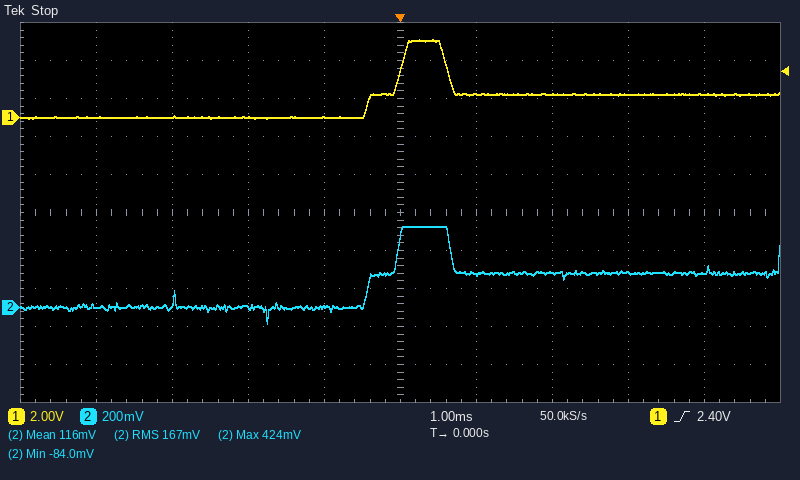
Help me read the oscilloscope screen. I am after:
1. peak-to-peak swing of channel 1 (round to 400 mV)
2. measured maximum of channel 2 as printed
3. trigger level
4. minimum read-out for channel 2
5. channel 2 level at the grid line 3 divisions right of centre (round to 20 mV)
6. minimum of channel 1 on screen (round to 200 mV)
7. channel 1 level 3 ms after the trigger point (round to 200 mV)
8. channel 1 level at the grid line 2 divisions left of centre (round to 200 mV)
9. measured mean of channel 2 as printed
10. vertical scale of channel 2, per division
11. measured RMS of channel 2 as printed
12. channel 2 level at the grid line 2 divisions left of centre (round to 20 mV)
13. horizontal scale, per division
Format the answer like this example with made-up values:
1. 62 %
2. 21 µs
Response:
1. 4.0 V
2. 424 mV
3. 2.40 V
4. -84.0 mV
5. 180 mV
6. 0.0 V
7. 1.2 V
8. 0.0 V
9. 116 mV
10. 200 mV
11. 167 mV
12. 0 mV
13. 1 ms
